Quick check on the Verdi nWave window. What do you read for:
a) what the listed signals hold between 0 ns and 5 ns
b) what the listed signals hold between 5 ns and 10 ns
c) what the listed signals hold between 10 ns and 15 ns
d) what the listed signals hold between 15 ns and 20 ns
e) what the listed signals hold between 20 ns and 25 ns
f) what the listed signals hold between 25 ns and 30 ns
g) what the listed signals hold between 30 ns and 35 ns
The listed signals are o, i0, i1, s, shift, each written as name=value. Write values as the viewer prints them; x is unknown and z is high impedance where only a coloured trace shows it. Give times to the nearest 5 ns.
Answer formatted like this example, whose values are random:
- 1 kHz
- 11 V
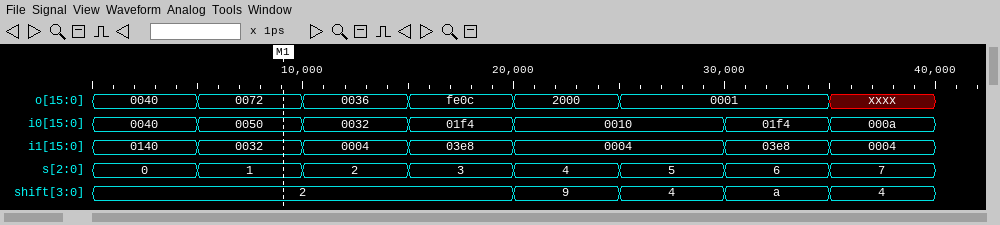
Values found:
- o=0040, i0=0040, i1=0140, s=0, shift=2
- o=0072, i0=0050, i1=0032, s=1, shift=2
- o=0036, i0=0032, i1=0004, s=2, shift=2
- o=fe0c, i0=01f4, i1=03e8, s=3, shift=2
- o=2000, i0=0010, i1=0004, s=4, shift=9
- o=0001, i0=0010, i1=0004, s=5, shift=4
- o=0001, i0=01f4, i1=03e8, s=6, shift=a
